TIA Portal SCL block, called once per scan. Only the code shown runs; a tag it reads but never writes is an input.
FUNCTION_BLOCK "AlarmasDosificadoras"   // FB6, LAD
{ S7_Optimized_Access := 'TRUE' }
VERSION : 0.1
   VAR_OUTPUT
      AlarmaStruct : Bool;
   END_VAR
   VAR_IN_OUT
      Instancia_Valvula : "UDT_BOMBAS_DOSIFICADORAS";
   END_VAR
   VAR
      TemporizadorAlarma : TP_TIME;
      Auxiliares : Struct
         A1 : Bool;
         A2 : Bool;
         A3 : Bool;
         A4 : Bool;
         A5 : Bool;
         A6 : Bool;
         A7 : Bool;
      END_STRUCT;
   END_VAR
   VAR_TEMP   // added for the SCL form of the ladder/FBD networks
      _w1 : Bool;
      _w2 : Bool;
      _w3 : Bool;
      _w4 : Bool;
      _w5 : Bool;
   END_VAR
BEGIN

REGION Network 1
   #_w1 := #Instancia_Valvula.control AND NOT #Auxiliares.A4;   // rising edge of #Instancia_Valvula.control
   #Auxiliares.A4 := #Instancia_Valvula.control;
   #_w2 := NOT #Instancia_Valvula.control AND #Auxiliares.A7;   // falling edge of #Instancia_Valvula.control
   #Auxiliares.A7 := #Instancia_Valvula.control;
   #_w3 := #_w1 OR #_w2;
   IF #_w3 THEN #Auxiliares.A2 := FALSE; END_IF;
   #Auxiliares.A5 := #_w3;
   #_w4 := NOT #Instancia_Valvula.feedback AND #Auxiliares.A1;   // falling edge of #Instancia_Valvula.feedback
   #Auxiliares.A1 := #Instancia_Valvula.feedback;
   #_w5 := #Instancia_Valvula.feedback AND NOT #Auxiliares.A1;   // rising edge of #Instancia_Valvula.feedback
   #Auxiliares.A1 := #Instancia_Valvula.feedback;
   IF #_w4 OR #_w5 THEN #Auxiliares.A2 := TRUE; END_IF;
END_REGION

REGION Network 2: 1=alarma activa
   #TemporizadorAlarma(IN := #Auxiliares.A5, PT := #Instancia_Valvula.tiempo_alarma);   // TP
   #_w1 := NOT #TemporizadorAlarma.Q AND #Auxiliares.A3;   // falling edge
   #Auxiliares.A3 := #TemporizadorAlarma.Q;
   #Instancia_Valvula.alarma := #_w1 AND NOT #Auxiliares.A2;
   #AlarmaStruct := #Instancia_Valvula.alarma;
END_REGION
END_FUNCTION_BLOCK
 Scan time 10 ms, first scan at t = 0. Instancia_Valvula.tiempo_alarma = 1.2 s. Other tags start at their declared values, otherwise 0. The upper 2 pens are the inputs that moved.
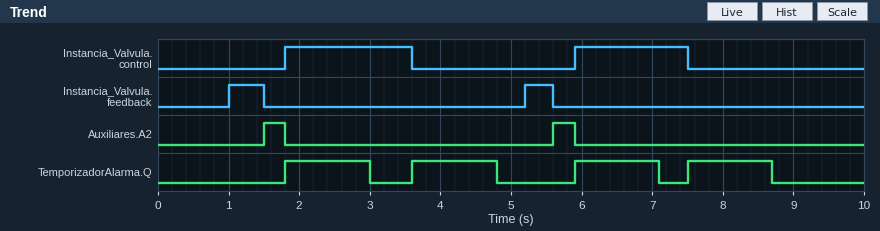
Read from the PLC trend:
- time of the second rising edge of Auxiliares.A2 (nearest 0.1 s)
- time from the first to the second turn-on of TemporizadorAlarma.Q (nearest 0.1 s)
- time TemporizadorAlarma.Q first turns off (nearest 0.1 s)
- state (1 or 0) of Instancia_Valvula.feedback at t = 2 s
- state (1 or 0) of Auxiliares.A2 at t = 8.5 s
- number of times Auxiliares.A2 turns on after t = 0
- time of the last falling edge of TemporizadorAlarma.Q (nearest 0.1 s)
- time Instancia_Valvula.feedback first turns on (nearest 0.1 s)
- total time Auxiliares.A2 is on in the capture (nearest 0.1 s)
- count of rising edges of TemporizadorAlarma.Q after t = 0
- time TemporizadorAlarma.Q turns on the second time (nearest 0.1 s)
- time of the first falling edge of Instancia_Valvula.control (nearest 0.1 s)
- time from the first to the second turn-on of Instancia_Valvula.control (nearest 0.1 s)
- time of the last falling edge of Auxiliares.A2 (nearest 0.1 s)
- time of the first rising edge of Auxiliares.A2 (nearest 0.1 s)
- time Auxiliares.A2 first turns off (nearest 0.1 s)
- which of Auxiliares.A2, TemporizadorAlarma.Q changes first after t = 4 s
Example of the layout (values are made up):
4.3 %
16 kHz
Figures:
5.6 s
1.8 s
3.0 s
0
0
2
8.7 s
1.0 s
0.6 s
4
3.6 s
3.6 s
4.1 s
5.9 s
1.5 s
1.8 s
TemporizadorAlarma.Q
